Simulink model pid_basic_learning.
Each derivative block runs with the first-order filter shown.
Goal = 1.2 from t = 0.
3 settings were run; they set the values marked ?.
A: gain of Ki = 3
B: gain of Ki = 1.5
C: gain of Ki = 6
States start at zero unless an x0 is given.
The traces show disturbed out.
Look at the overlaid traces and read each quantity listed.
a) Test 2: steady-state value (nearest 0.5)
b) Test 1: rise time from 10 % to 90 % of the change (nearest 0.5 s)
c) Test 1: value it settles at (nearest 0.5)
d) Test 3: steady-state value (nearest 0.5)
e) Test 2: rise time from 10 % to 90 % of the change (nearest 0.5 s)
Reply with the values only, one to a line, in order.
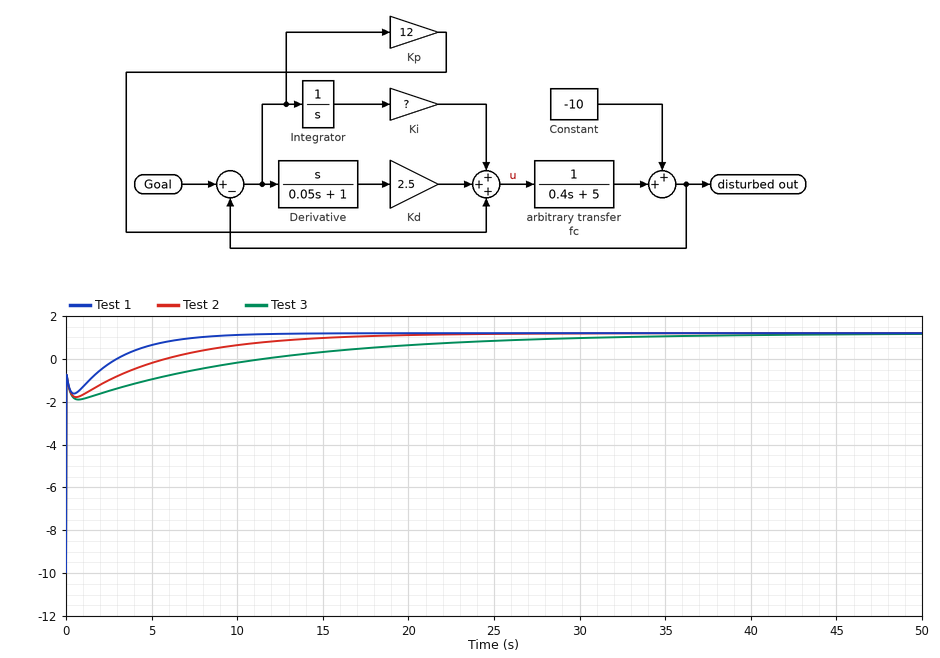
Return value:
1.0
3.0 s
1.0
1.0
6.0 s
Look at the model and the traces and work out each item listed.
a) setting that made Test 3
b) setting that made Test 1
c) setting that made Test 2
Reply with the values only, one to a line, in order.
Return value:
B
C
A
